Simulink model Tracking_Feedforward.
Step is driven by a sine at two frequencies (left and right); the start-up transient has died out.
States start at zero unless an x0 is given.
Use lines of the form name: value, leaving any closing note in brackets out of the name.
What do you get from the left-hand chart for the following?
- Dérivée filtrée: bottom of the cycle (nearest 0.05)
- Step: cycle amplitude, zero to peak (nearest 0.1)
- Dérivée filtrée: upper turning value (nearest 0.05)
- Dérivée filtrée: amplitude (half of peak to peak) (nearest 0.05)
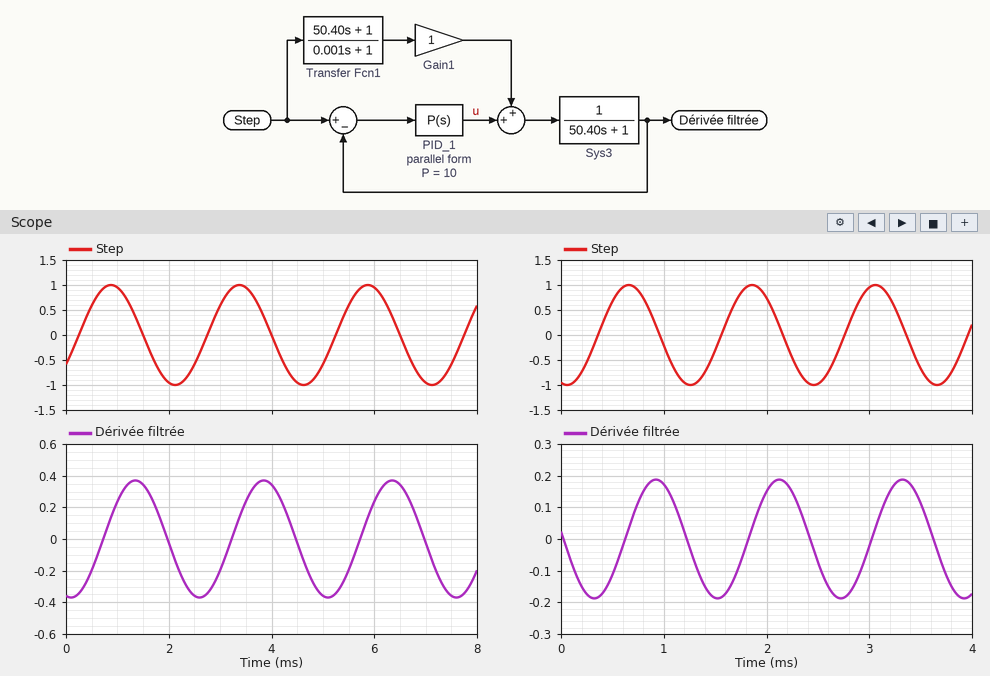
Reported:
Dérivée filtrée: bottom of the cycle: -0.35
Step: cycle amplitude, zero to peak: 1.0
Dérivée filtrée: upper turning value: 0.35
Dérivée filtrée: amplitude (half of peak to peak): 0.35
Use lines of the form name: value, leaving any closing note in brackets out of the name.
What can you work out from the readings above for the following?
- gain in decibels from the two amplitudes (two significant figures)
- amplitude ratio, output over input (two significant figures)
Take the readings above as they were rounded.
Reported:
gain in decibels from the two amplitudes: -9.1 dB
amplitude ratio, output over input: 0.35
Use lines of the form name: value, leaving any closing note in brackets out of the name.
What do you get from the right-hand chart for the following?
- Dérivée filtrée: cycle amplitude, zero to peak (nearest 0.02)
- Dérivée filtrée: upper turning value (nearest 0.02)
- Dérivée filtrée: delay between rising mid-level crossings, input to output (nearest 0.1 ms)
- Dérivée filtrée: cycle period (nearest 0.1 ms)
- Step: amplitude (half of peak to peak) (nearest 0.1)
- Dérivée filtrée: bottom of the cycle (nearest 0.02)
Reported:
Dérivée filtrée: cycle amplitude, zero to peak: 0.18
Dérivée filtrée: upper turning value: 0.18
Dérivée filtrée: delay between rising mid-level crossings, input to output: 0.3 ms
Dérivée filtrée: cycle period: 1.2 ms
Step: amplitude (half of peak to peak): 1.0
Dérivée filtrée: bottom of the cycle: -0.18
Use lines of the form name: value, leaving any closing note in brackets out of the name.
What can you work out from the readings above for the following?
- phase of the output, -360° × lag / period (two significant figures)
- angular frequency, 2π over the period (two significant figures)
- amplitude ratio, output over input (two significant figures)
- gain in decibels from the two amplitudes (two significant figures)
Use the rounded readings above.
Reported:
phase of the output, -360° × lag / period: -90°
angular frequency, 2π over the period: 5.2 rad/ms
amplitude ratio, output over input: 0.18
gain in decibels from the two amplitudes: -15 dB
